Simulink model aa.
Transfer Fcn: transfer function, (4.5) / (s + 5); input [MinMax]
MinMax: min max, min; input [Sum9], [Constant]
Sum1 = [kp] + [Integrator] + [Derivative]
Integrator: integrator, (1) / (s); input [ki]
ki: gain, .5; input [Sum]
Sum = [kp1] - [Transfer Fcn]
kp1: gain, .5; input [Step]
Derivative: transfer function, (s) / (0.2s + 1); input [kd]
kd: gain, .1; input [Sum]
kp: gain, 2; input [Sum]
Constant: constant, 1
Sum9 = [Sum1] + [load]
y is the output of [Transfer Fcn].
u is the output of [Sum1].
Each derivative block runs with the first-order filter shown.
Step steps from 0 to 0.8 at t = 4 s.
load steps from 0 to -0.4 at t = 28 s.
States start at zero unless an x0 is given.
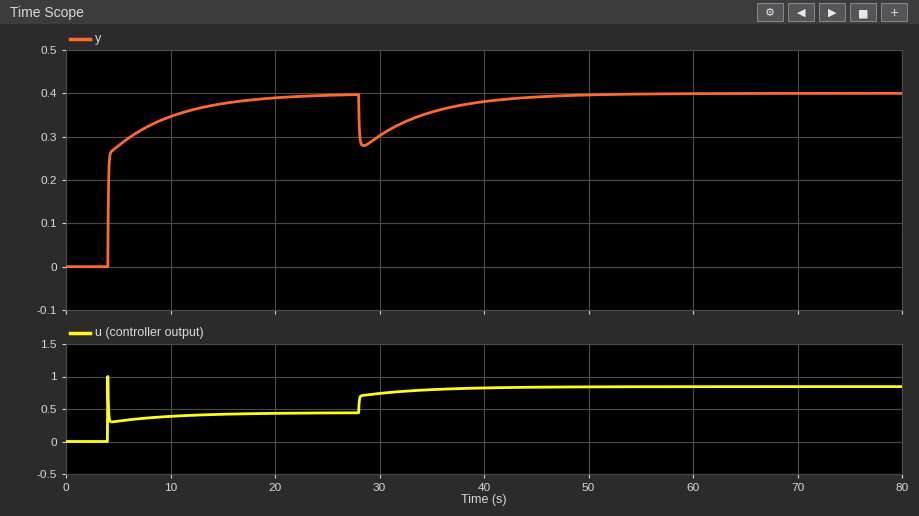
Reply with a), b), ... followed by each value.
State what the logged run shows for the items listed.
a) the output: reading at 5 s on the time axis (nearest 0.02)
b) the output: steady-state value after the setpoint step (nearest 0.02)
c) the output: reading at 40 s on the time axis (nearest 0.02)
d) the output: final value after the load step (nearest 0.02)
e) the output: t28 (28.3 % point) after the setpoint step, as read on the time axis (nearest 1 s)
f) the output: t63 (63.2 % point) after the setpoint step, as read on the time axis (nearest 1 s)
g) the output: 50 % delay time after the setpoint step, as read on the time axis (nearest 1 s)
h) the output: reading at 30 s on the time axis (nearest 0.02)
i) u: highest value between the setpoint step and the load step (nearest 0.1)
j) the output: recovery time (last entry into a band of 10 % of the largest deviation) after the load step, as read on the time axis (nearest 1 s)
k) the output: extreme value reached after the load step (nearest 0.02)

a) 0.28
b) 0.40
c) 0.38
d) 0.40
e) 4 s
f) 4 s
g) 4 s
h) 0.30
i) 1.0
j) 43 s
k) 0.28
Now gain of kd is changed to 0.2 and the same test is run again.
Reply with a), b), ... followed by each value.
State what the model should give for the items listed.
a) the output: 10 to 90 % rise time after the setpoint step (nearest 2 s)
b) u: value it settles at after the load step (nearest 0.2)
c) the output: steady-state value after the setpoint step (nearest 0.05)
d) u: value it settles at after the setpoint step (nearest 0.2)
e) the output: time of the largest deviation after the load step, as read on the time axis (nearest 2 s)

a) 8 s
b) 0.8
c) 0.40
d) 0.4
e) 28 s
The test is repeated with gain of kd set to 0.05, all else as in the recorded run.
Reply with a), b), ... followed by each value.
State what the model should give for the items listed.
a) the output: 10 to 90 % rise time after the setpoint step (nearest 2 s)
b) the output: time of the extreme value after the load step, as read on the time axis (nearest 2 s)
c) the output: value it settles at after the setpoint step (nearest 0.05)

a) 8 s
b) 28 s
c) 0.40
